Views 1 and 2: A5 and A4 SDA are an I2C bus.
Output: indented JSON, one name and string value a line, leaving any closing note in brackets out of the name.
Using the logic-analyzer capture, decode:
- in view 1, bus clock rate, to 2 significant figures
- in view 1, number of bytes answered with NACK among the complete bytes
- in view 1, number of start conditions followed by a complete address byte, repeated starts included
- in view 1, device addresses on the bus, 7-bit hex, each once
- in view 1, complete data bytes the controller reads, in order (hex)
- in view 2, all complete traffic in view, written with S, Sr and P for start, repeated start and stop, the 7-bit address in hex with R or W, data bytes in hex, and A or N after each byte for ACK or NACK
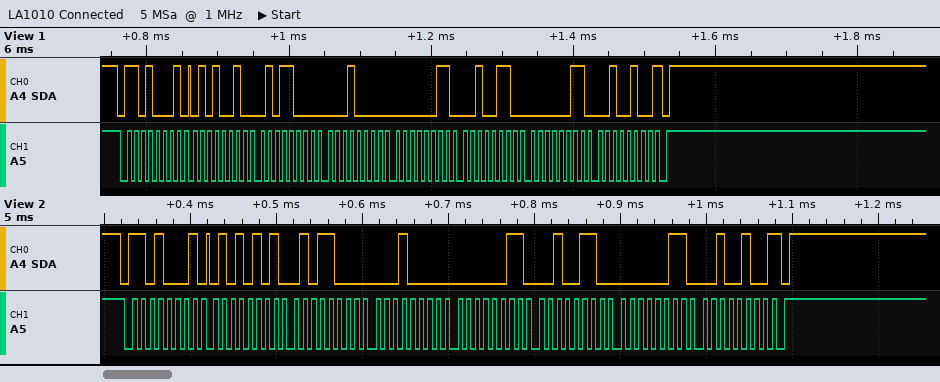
{
  "in view 1, bus clock rate, to 2 significant figures": "100 kHz",
  "in view 1, number of bytes answered with NACK among the complete bytes": "1",
  "in view 1, number of start conditions followed by a complete address byte, repeated starts included": "1",
  "in view 1, device addresses on the bus, 7-bit hex, each once": "0x68",
  "in view 1, complete data bytes the controller reads, in order": "52 58 10 03 26 03 24",
  "in view 2, all complete traffic in view, written with S, Sr and P for start, repeated start and stop, the 7-bit address in hex with R or W, data bytes in hex, and A or N after each byte for ACK or NACK": "S 68R A 55 A 58 A 10 A 03 A 26 A 03 A 24 N P"
}
